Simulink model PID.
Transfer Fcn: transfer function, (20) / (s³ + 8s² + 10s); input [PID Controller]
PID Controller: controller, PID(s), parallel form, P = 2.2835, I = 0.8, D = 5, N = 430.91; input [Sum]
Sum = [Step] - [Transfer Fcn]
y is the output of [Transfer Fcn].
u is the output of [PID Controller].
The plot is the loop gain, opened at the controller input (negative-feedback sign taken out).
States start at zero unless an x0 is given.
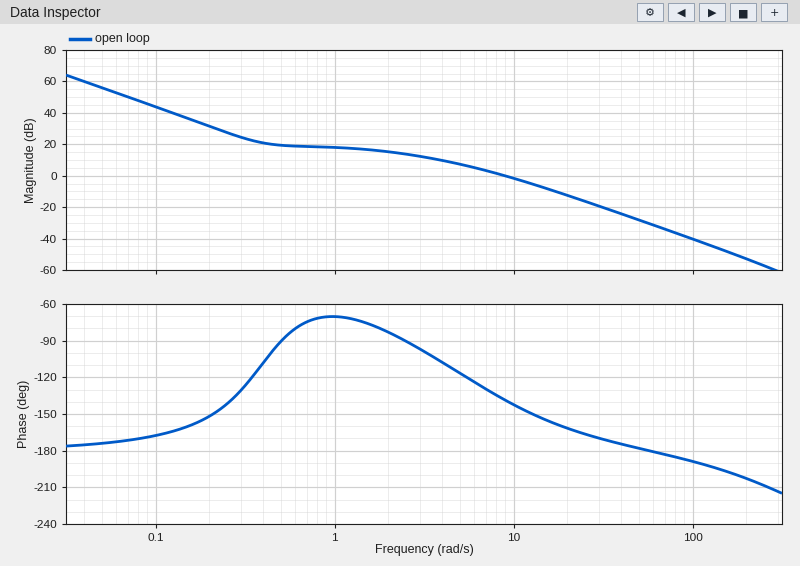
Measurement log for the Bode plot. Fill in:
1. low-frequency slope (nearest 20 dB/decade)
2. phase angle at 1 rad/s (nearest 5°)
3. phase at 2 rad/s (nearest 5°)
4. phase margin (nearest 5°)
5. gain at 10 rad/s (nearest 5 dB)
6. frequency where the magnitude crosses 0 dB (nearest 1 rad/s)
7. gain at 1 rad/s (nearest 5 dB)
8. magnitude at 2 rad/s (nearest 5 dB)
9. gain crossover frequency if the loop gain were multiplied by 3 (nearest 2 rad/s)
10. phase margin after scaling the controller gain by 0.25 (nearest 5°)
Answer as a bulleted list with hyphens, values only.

- -40 dB/decade
- -70°
- -85°
- 40°
- 0 dB
- 9 rad/s
- 20 dB
- 15 dB
- 16 rad/s
- 80°
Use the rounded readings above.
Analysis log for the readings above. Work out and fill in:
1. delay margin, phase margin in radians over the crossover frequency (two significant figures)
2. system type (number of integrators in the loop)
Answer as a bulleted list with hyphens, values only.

- 0.078 s
- 2
